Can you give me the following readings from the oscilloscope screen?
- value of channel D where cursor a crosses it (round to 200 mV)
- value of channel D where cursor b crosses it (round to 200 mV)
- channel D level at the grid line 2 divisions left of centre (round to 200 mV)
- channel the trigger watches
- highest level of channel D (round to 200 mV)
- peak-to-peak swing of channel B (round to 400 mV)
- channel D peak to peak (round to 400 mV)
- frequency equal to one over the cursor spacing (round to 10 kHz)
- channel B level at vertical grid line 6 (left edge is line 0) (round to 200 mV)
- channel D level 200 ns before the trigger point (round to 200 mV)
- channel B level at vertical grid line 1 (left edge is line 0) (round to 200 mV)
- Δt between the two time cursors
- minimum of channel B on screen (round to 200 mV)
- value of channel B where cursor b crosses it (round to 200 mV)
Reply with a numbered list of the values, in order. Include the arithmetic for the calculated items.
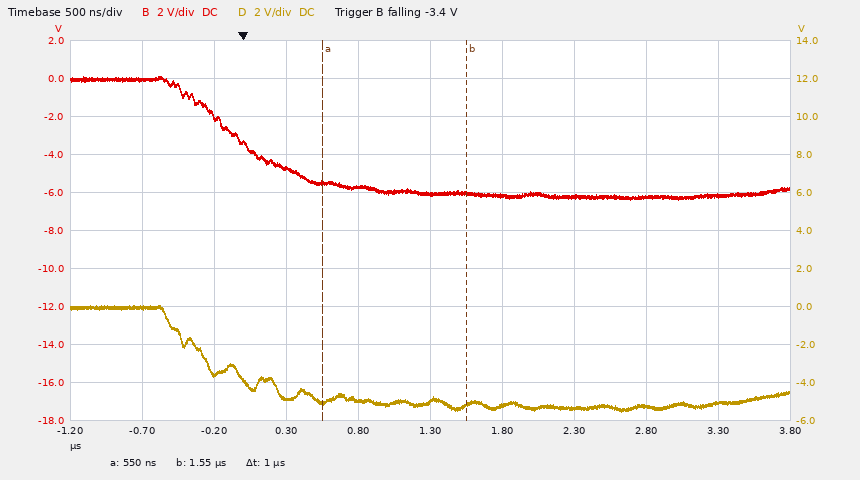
1. -5.0 V
2. -5.2 V
3. -4.8 V
4. channel B
5. 0.0 V
6. 6.4 V
7. 5.6 V
8. 1 / 1 µs ≈ 1.00 MHz
9. -6.2 V
10. -3.6 V
11. 0.0 V
12. 1 µs
13. -6.4 V
14. -6.0 V
